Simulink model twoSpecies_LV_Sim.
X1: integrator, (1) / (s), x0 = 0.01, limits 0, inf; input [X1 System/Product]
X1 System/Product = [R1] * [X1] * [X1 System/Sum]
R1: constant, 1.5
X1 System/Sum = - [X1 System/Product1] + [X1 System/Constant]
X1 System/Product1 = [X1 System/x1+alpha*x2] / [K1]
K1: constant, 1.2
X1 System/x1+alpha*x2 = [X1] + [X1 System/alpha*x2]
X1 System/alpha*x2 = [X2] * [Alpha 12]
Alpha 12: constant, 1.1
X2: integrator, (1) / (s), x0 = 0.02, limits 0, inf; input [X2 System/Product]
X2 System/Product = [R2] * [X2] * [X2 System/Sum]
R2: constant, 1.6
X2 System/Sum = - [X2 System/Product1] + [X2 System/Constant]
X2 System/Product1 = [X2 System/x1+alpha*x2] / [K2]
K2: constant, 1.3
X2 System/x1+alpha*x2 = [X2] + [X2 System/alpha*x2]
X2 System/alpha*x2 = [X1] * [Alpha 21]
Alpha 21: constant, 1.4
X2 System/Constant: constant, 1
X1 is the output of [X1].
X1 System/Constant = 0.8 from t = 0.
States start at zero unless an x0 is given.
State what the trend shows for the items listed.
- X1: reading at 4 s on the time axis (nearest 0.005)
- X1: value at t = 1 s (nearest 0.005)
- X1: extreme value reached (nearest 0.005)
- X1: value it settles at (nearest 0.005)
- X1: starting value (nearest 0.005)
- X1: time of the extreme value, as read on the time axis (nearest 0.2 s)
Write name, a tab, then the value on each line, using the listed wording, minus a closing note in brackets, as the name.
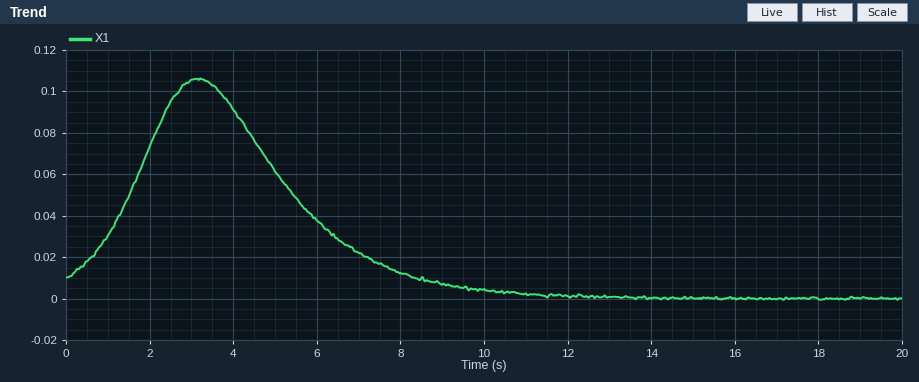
X1: reading at 4 s on the time axis	0.090
X1: value at t = 1 s	0.030
X1: extreme value reached	0.105
X1: value it settles at	0.000
X1: starting value	0.010
X1: time of the extreme value, as read on the time axis	3.2 s
